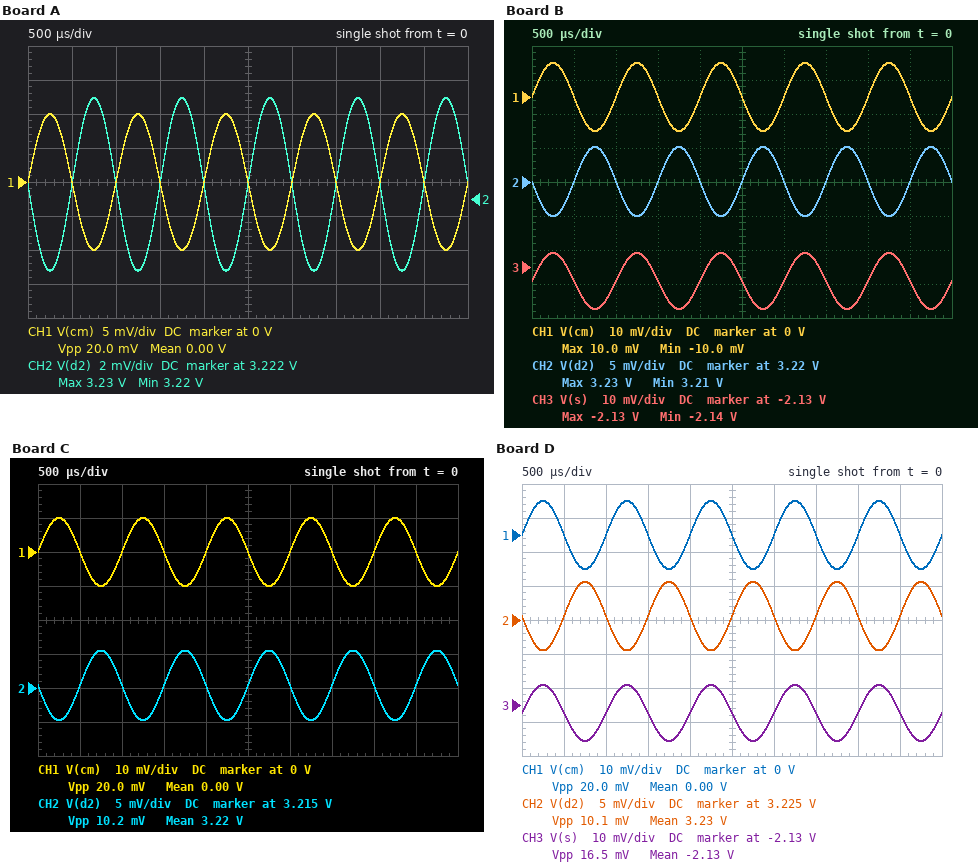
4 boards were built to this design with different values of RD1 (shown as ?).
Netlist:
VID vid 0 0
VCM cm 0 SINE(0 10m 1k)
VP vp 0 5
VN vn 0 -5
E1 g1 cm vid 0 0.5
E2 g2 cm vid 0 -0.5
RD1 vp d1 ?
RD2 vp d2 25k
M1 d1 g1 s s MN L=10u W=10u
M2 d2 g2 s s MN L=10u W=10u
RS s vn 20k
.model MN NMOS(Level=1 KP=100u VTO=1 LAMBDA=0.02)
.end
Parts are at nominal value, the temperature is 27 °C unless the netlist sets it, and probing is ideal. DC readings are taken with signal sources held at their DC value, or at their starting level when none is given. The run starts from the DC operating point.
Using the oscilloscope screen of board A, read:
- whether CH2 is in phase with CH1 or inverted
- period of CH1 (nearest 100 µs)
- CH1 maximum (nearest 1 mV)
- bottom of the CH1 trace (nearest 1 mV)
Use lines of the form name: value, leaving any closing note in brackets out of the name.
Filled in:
whether CH2 is in phase with CH1 or inverted: inverted
period of CH1: 1.0 ms
CH1 maximum: 10 mV
bottom of the CH1 trace: -10 mV
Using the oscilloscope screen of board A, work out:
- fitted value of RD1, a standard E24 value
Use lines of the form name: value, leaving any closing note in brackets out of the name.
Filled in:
fitted value of RD1, a standard E24 value: 12 kΩ
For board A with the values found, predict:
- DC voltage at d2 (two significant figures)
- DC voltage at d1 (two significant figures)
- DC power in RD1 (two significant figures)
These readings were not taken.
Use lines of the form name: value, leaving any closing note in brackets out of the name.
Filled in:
DC voltage at d2: 3.2 V
DC voltage at d1: 4.1 V
DC power in RD1: 63 µW
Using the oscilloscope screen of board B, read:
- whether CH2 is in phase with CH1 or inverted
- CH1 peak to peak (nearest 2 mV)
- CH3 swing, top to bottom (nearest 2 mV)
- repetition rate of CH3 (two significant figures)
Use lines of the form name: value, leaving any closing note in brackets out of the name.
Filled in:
whether CH2 is in phase with CH1 or inverted: inverted
CH1 peak to peak: 20 mV
CH3 swing, top to bottom: 16 mV
repetition rate of CH3: 1.0 kHz
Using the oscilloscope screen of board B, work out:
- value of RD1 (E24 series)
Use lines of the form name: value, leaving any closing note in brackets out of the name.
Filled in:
value of RD1: 15 kΩ
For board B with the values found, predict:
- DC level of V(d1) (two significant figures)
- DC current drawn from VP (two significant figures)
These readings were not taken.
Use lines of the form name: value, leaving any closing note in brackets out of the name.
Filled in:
DC level of V(d1): 3.9 V
DC current drawn from VP: 140 µA
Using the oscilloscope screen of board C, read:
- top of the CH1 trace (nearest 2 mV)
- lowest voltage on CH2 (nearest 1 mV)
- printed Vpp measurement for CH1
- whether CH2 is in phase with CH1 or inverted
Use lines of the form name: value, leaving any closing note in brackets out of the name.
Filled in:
top of the CH1 trace: 10 mV
lowest voltage on CH2: 3.210 V
printed Vpp measurement for CH1: 20.0 mV
whether CH2 is in phase with CH1 or inverted: inverted
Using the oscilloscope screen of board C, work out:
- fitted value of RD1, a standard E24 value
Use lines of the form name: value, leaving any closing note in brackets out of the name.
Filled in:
fitted value of RD1, a standard E24 value: 20 kΩ
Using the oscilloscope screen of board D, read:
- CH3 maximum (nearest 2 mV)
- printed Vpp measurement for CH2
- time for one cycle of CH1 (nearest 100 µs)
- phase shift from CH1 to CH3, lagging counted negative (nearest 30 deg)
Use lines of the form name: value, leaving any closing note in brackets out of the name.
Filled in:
CH3 maximum: -2.124 V
printed Vpp measurement for CH2: 10.1 mV
time for one cycle of CH1: 1.0 ms
phase shift from CH1 to CH3, lagging counted negative: 0 deg
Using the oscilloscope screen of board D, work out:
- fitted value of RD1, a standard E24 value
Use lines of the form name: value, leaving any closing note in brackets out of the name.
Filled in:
fitted value of RD1, a standard E24 value: 9.1 kΩ
